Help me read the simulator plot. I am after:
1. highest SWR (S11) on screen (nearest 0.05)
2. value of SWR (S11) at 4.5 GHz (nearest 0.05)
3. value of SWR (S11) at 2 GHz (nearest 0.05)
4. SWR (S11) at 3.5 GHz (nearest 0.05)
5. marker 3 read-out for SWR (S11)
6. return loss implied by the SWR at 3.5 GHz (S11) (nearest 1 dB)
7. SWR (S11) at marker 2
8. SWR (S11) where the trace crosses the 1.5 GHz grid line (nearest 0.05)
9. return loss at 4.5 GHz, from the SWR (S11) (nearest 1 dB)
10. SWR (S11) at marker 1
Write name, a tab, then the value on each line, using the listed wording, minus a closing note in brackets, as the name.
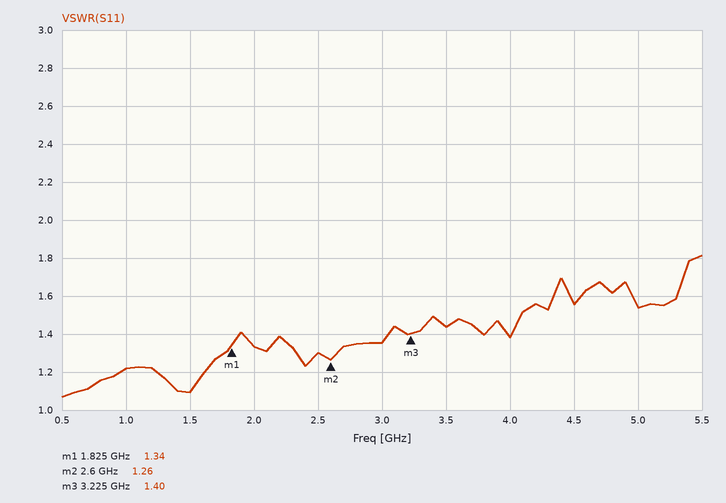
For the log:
highest SWR (S11) on screen	1.80
value of SWR (S11) at 4.5 GHz	1.55
value of SWR (S11) at 2 GHz	1.35
SWR (S11) at 3.5 GHz	1.45
marker 3 read-out for SWR	1.40
return loss implied by the SWR at 3.5 GHz (S11)	15 dB
SWR (S11) at marker 2	1.26
SWR (S11) where the trace crosses the 1.5 GHz grid line	1.10
return loss at 4.5 GHz, from the SWR (S11)	13 dB
SWR (S11) at marker 1	1.34
